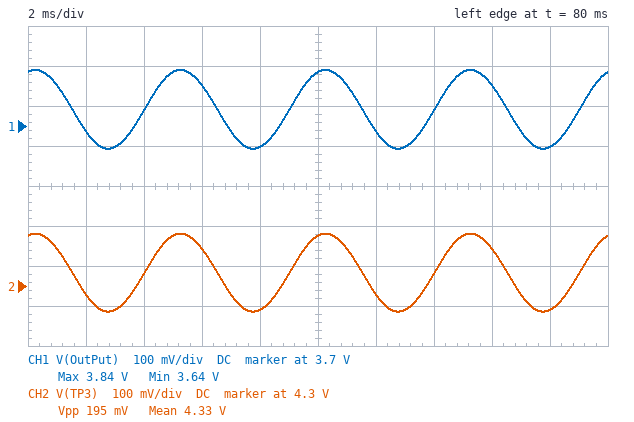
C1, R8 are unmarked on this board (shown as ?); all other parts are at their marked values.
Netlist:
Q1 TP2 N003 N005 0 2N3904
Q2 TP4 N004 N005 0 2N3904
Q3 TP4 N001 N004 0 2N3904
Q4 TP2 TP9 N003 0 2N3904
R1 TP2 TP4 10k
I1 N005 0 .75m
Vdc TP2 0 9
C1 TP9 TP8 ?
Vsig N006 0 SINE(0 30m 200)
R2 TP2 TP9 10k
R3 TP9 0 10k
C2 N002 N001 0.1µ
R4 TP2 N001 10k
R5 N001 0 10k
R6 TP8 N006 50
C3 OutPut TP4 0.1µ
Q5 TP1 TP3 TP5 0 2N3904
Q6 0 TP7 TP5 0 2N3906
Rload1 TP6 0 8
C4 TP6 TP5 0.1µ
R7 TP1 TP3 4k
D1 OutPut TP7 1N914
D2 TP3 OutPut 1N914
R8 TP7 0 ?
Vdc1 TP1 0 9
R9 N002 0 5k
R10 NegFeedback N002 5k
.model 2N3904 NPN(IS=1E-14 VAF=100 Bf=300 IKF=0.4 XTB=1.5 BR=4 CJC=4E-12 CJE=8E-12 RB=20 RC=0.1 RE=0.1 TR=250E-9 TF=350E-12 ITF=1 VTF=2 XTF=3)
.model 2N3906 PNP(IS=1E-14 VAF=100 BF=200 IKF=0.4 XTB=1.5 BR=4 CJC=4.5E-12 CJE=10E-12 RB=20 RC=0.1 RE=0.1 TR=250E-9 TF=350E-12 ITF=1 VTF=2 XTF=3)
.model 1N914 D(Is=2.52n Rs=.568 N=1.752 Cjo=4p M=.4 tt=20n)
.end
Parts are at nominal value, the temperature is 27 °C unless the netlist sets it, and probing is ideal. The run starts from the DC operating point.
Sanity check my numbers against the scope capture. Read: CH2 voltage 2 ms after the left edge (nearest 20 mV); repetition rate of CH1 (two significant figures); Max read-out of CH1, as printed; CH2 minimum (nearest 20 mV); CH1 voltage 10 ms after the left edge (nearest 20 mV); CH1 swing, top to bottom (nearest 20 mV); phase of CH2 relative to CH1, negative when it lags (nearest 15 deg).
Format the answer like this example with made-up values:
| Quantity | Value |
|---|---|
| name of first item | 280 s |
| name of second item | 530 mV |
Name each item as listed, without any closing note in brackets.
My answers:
| Quantity | Value |
|---|---|
| CH2 voltage 2 ms after the left edge | 4.28 V |
| repetition rate of CH1 | 200 Hz |
| Max read-out of CH1, as printed | 3.84 V |
| CH2 minimum | 4.24 V |
| CH1 voltage 10 ms after the left edge | 3.84 V |
| CH1 swing, top to bottom | 200 mV |
| phase of CH2 relative to CH1, negative when it lags | 0 deg |
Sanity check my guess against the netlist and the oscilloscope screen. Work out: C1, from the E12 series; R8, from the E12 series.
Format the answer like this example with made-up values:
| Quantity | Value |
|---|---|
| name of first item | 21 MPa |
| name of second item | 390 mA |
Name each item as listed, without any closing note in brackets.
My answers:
| Quantity | Value |
|---|---|
| C1, from the E12 series | 220 nF |
| R8, from the E12 series | 2.7 kΩ |
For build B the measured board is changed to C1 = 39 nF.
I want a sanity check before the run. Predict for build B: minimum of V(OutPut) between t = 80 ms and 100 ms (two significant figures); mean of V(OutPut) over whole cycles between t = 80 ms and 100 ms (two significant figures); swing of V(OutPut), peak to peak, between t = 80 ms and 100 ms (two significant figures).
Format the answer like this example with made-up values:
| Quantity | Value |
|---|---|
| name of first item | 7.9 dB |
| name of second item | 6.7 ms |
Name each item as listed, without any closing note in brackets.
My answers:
| Quantity | Value |
|---|---|
| minimum of V(OutPut) between t = 80 ms and 100 ms | 3.7 V |
| mean of V(OutPut) over whole cycles between t = 80 ms and 100 ms | 3.7 V |
| swing of V(OutPut), peak to peak, between t = 80 ms and 100 ms | 59 mV |
